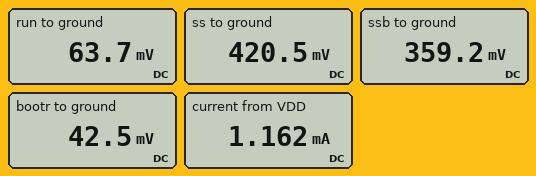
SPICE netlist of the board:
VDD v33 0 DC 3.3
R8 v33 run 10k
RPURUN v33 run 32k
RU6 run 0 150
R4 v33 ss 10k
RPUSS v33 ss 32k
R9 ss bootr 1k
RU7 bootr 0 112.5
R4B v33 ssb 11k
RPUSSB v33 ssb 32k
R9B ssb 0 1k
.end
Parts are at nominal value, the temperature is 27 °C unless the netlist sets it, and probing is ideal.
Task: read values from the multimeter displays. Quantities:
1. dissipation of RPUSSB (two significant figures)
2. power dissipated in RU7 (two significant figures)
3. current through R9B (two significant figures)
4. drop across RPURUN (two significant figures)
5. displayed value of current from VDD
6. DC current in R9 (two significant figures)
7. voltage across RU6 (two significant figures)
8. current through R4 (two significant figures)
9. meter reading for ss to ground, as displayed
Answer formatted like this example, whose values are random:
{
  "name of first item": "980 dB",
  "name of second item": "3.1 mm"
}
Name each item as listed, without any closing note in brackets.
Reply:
{
  "dissipation of RPUSSB": "270 µW",
  "power dissipated in RU7": "16 µW",
  "current through R9B": "360 µA",
  "drop across RPURUN": "3.2 V",
  "displayed value of current from VDD": "1.162 mA",
  "DC current in R9": "380 µA",
  "voltage across RU6": "64 mV",
  "current through R4": "290 µA",
  "meter reading for ss to ground, as displayed": "420.5 mV"
}
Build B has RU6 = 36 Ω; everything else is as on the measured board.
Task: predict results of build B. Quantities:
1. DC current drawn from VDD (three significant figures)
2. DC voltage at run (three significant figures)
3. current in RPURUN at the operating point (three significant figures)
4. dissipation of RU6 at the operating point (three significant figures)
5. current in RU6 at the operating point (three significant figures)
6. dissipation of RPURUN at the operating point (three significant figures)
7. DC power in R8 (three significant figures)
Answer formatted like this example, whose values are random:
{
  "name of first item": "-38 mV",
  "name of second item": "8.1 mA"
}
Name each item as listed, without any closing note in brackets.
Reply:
{
  "DC current drawn from VDD": "1.17 mA",
  "DC voltage at run": "15.5 mV",
  "current in RPURUN at the operating point": "103 µA",
  "dissipation of RU6 at the operating point": "6.69 µW",
  "current in RU6 at the operating point": "431 µA",
  "dissipation of RPURUN at the operating point": "337 µW",
  "DC power in R8": "1.08 mW"
}
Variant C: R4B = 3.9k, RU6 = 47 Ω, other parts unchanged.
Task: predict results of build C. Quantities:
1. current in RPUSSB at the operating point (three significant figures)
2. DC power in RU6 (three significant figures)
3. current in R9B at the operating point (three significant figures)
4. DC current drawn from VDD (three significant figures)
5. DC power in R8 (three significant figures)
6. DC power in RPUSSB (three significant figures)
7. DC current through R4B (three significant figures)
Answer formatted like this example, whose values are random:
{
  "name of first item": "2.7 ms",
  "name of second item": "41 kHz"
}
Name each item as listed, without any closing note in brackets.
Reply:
{
  "current in RPUSSB at the operating point": "80.1 µA",
  "DC power in RU6": "8.71 µW",
  "current in R9B at the operating point": "737 µA",
  "DC current drawn from VDD": "1.55 mA",
  "DC power in R8": "1.08 mW",
  "DC power in RPUSSB": "205 µW",
  "DC current through R4B": "657 µA"
}
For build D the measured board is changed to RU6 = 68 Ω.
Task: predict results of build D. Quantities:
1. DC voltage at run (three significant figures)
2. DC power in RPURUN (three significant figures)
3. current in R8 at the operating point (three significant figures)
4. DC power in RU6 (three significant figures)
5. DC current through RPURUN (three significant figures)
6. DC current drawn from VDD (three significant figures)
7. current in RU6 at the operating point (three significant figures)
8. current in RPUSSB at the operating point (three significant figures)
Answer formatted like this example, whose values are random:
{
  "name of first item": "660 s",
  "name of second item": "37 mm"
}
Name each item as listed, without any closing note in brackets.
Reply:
{
  "DC voltage at run": "29.2 mV",
  "DC power in RPURUN": "334 µW",
  "current in R8 at the operating point": "327 µA",
  "DC power in RU6": "12.5 µW",
  "DC current through RPURUN": "102 µA",
  "DC current drawn from VDD": "1.17 mA",
  "current in RU6 at the operating point": "429 µA",
  "current in RPUSSB at the operating point": "91.9 µA"
}
